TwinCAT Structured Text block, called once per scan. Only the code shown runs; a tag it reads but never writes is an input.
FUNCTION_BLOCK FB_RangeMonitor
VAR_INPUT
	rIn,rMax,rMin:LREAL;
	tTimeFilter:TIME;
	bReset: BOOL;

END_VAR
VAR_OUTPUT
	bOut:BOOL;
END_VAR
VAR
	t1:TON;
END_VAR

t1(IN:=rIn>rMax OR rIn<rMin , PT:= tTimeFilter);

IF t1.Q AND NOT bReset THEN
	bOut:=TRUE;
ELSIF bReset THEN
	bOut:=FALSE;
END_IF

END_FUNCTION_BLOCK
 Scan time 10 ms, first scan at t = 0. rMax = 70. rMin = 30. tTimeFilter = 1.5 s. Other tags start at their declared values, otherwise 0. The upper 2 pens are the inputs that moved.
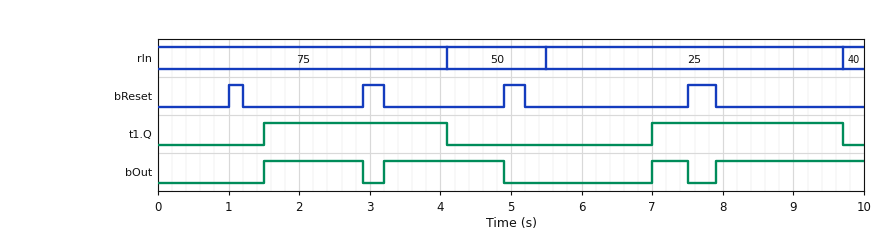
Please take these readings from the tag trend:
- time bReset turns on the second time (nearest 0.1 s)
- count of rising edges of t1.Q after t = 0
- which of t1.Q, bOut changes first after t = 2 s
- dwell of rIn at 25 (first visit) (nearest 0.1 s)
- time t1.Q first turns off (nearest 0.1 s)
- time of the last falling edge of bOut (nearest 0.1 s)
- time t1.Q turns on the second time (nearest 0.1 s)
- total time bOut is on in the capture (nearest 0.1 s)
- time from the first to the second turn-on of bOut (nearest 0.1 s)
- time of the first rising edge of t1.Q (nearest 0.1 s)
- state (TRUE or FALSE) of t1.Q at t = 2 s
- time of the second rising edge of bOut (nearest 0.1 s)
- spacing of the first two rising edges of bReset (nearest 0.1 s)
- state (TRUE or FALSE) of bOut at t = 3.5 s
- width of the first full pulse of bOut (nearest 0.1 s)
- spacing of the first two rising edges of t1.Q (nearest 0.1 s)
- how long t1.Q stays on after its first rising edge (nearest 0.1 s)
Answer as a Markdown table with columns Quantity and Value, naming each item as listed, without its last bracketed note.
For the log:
| Quantity | Value |
|---|---|
| time bReset turns on the second time | 2.9 s |
| count of rising edges of t1.Q after t = 0 | 2 |
| which of t1.Q, bOut changes first after t = 2 s | bOut |
| dwell of rIn at 25 (first visit) | 4.2 s |
| time t1.Q first turns off | 4.1 s |
| time of the last falling edge of bOut | 7.5 s |
| time t1.Q turns on the second time | 7.0 s |
| total time bOut is on in the capture | 5.7 s |
| time from the first to the second turn-on of bOut | 1.7 s |
| time of the first rising edge of t1.Q | 1.5 s |
| state (TRUE or FALSE) of t1.Q at t = 2 s | TRUE |
| time of the second rising edge of bOut | 3.2 s |
| spacing of the first two rising edges of bReset | 1.9 s |
| state (TRUE or FALSE) of bOut at t = 3.5 s | TRUE |
| width of the first full pulse of bOut | 1.4 s |
| spacing of the first two rising edges of t1.Q | 5.5 s |
| how long t1.Q stays on after its first rising edge | 2.6 s |
